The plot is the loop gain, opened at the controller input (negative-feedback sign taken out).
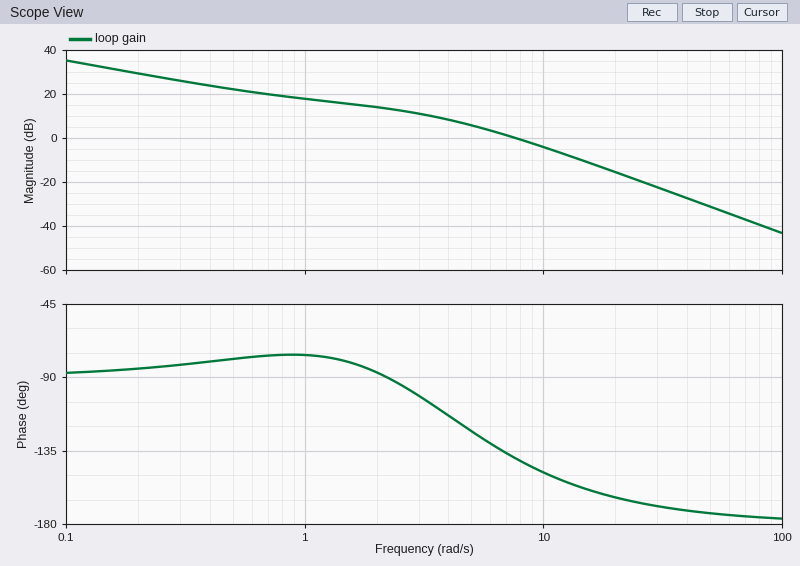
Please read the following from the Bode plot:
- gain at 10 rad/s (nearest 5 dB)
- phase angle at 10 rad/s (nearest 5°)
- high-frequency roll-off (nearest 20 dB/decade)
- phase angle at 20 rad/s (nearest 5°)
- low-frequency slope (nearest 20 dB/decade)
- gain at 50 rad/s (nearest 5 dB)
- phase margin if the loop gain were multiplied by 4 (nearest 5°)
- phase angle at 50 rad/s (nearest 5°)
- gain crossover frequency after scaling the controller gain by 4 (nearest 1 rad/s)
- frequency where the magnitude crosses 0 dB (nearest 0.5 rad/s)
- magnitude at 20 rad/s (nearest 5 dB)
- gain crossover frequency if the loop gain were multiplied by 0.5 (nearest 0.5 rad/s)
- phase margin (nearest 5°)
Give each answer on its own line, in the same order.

-5 dB
-150°
-40 dB/decade
-165°
-20 dB/decade
-30 dB
20°
-175°
16 rad/s
7.5 rad/s
-15 dB
5.0 rad/s
40°
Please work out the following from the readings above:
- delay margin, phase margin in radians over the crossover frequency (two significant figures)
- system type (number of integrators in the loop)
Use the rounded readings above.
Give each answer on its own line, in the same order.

0.093 s
1
